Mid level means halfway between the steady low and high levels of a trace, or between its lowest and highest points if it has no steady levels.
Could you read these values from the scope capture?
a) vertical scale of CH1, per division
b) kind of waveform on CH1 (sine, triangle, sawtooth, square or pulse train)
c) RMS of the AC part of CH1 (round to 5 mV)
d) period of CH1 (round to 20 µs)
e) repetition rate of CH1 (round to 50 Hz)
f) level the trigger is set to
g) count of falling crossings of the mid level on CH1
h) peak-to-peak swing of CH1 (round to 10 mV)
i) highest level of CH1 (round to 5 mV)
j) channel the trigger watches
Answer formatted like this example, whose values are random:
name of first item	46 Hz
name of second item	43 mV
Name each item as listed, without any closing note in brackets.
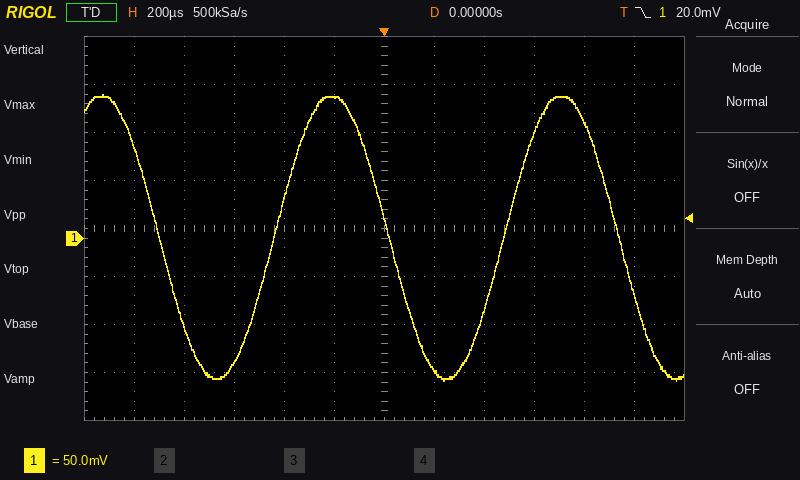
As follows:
vertical scale of CH1, per division	50 mV
kind of waveform on CH1	sine
RMS of the AC part of CH1	105 mV
period of CH1	920 µs
repetition rate of CH1	1.10 kHz
level the trigger is set to	20.0 mV
count of falling crossings of the mid level on CH1	3
peak-to-peak swing of CH1	300 mV
highest level of CH1	150 mV
channel the trigger watches	CH1
